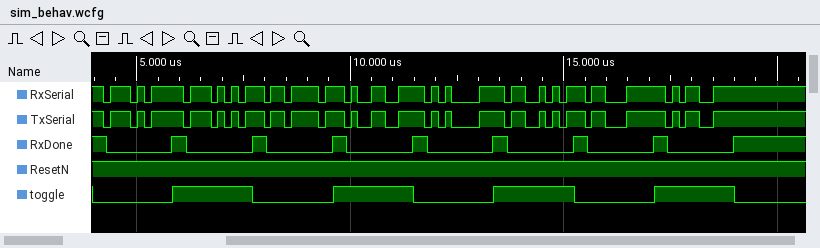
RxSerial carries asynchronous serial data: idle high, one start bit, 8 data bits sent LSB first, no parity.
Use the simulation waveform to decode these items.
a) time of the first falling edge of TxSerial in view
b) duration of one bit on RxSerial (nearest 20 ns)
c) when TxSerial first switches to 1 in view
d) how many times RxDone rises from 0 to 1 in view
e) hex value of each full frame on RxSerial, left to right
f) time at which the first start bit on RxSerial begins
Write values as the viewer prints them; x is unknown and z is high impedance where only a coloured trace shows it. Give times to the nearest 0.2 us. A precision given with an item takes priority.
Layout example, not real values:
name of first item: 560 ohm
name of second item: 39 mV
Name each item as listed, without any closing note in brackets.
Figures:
time of the first falling edge of TxSerial in view: 4.2 us
duration of one bit on RxSerial: 160 ns
when TxSerial first switches to 1 in view: 4.4 us
how many times RxDone rises from 0 to 1 in view: 8
hex value of each full frame on RxSerial, left to right: D7, 57, 7B, 99, 85, 53, E3, CD
time at which the first start bit on RxSerial begins: 4.2 us
